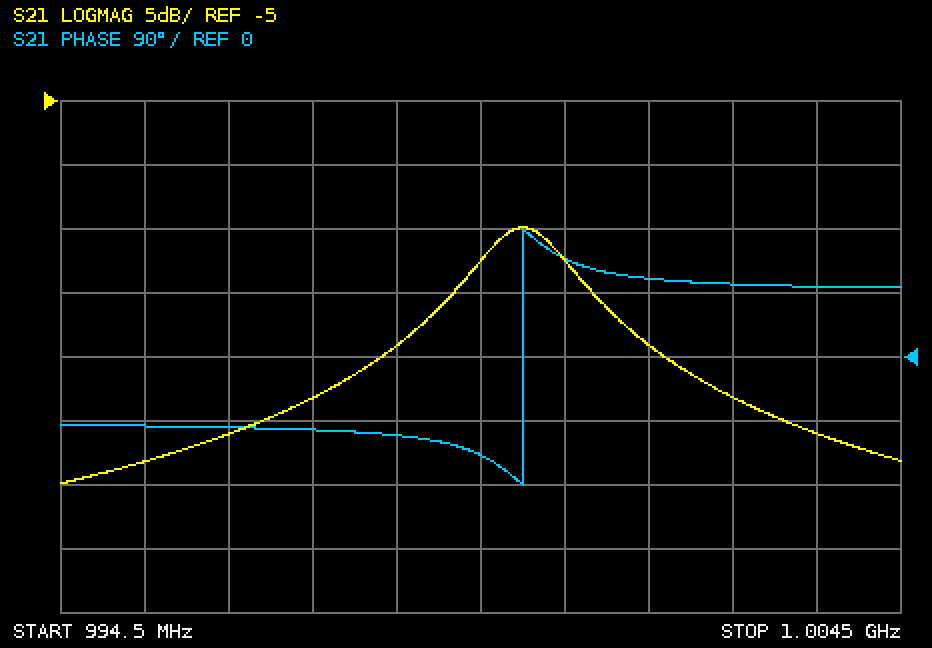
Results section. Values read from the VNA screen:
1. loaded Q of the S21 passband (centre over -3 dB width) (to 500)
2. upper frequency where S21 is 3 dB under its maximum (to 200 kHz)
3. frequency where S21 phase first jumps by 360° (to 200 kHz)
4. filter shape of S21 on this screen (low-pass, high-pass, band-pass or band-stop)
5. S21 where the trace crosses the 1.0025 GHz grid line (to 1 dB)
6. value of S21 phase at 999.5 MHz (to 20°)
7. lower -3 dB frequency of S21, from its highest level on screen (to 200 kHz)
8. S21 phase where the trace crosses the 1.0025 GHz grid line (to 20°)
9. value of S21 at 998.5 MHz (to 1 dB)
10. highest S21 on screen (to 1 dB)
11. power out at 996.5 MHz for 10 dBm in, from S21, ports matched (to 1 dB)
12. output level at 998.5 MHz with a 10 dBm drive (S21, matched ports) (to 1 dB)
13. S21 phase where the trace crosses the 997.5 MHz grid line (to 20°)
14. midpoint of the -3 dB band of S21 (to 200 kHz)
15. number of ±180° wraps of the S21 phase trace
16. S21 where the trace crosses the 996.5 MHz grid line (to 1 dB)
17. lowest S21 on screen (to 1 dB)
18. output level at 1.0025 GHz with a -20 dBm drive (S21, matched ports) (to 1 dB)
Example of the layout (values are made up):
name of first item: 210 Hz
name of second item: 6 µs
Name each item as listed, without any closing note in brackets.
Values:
loaded Q of the S21 passband (centre over -3 dB width): 1000
upper frequency where S21 is 3 dB under its maximum: 1.0006 GHz
frequency where S21 phase first jumps by 360°: 1.0000 GHz
filter shape of S21 on this screen: band-pass
S21 where the trace crosses the 1.0025 GHz grid line: -28 dB
value of S21 phase at 999.5 MHz: -140°
lower -3 dB frequency of S21, from its highest level on screen: 999.4 MHz
S21 phase where the trace crosses the 1.0025 GHz grid line: 100°
value of S21 at 998.5 MHz: -24 dB
highest S21 on screen: -15 dB
power out at 996.5 MHz for 10 dBm in, from S21, ports matched: -21 dBm
output level at 998.5 MHz with a 10 dBm drive (S21, matched ports): -14 dBm
S21 phase where the trace crosses the 997.5 MHz grid line: -100°
midpoint of the -3 dB band of S21: 1.0000 GHz
number of ±180° wraps of the S21 phase trace: 1
S21 where the trace crosses the 996.5 MHz grid line: -31 dB
lowest S21 on screen: -35 dB
output level at 1.0025 GHz with a -20 dBm drive (S21, matched ports): -48 dBm
